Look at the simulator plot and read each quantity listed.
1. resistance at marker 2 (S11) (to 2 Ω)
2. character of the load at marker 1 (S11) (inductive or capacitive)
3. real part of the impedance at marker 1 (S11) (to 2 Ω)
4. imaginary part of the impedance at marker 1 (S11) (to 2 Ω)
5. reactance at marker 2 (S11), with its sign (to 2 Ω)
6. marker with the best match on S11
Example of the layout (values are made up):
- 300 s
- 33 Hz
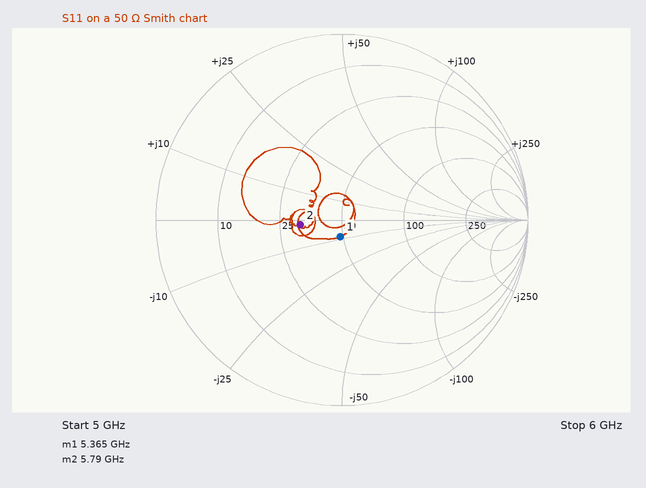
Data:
- 32 Ω
- capacitive
- 48 Ω
- -8 Ω
- -2 Ω
- marker 1
